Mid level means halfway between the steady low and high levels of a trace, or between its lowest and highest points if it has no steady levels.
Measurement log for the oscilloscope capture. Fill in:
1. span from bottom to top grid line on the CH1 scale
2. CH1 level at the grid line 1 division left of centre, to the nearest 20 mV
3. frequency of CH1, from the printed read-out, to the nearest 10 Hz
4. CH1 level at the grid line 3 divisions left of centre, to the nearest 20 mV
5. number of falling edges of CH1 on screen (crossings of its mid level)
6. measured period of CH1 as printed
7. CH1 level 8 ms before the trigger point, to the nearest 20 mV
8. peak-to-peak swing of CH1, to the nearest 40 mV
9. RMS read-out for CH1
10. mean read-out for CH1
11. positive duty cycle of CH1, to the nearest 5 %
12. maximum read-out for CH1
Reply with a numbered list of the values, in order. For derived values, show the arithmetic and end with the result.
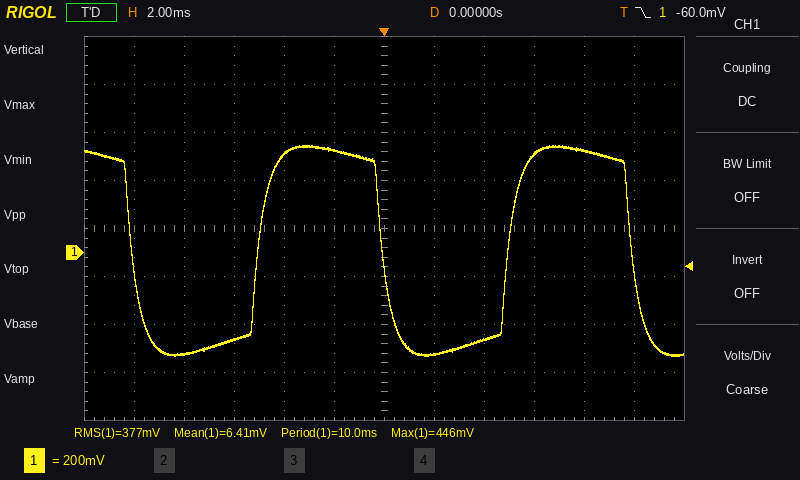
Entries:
1. 1.6 V
2. 420 mV
3. 1 / 10.0 ms ≈ 100 Hz
4. -360 mV
5. 3
6. 10.0 ms
7. -420 mV
8. 880 mV
9. 377 mV
10. 6.41 mV
11. 50 %
12. 446 mV
